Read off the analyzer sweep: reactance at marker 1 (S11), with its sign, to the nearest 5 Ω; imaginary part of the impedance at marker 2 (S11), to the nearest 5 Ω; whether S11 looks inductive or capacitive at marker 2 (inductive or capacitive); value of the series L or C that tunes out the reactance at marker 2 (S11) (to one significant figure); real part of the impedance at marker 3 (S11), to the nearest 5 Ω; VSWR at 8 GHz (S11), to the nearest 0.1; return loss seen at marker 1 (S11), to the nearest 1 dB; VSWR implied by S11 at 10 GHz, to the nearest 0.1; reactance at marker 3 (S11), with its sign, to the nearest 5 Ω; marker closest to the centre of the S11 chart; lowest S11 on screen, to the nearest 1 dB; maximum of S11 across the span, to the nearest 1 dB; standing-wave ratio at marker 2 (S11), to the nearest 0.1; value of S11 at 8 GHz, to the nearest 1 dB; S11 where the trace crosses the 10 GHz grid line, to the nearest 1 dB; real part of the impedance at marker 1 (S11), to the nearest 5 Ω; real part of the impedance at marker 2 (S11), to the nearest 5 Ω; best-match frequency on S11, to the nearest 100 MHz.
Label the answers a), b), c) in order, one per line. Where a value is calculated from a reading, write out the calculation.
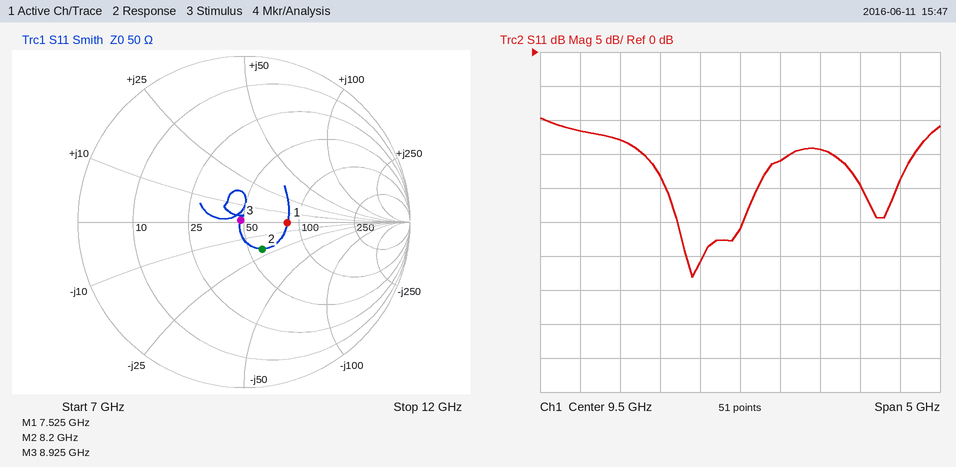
a) 0 Ω
b) -20 Ω
c) capacitive
d) L = 20 Ω/(2π × 8.2 GHz) ≈ 388 pH, so 400 pH to one significant figure
e) 50 Ω
f) |Γ| = 10^(-13/20) = 0.2239; VSWR = (1 + 0.2239)/(1 − 0.2239) ≈ 1.6
g) 12 dB
h) |Γ| = 10^(-16/20) = 0.1585; VSWR = (1 + 0.1585)/(1 − 0.1585) ≈ 1.4
i) 0 Ω
j) marker 3
k) -33 dB
l) -10 dB
m) 1.5
n) -13 dB
o) -16 dB
p) 85 Ω
q) 60 Ω
r) 8.9 GHz
